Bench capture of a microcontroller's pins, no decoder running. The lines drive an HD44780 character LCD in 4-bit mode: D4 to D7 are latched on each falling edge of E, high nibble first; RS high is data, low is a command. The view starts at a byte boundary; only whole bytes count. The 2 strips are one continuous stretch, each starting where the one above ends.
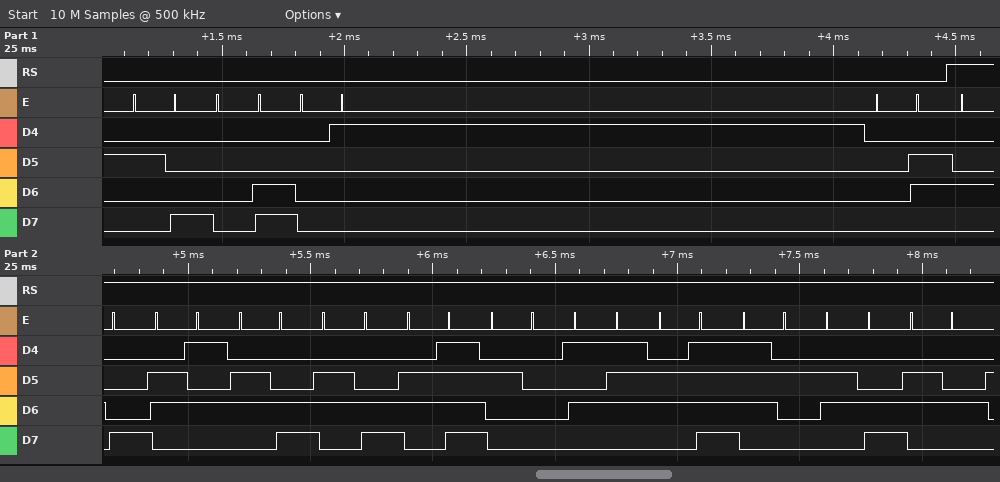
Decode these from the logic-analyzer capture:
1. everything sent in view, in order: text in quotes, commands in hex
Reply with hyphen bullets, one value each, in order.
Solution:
- 0x28 0x0C 0x01 0x06 "Hello World"
